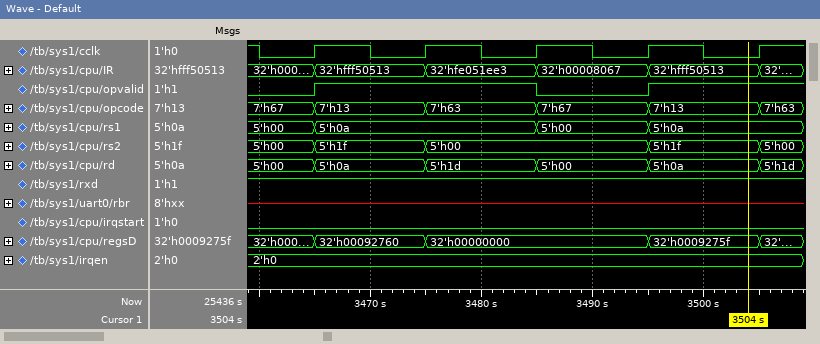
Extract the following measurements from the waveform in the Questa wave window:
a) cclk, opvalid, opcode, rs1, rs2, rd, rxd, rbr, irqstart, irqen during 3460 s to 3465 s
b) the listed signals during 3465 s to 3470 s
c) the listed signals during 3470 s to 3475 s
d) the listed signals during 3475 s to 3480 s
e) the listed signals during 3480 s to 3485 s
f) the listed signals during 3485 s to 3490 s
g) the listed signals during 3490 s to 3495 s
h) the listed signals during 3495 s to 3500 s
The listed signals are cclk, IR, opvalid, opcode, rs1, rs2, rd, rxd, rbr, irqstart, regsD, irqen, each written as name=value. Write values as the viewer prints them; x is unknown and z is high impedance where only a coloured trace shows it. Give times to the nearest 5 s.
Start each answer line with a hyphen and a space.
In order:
- cclk=0, opvalid=0, opcode=7'h67, rs1=5'h00, rs2=5'h00, rd=5'h00, rxd=1, rbr=x, irqstart=0, irqen=2'h0
- cclk=1, IR=32'hfff50513, opvalid=1, opcode=7'h13, rs1=5'h0a, rs2=5'h1f, rd=5'h0a, rxd=1, rbr=x, irqstart=0, regsD=32'h00092760, irqen=2'h0
- cclk=0, IR=32'hfff50513, opvalid=1, opcode=7'h13, rs1=5'h0a, rs2=5'h1f, rd=5'h0a, rxd=1, rbr=x, irqstart=0, regsD=32'h00092760, irqen=2'h0
- cclk=1, IR=32'hfe051ee3, opvalid=1, opcode=7'h63, rs1=5'h0a, rs2=5'h00, rd=5'h1d, rxd=1, rbr=x, irqstart=0, regsD=32'h00000000, irqen=2'h0
- cclk=0, IR=32'hfe051ee3, opvalid=1, opcode=7'h63, rs1=5'h0a, rs2=5'h00, rd=5'h1d, rxd=1, rbr=x, irqstart=0, regsD=32'h00000000, irqen=2'h0
- cclk=1, IR=32'h00008067, opvalid=0, opcode=7'h67, rs1=5'h00, rs2=5'h00, rd=5'h00, rxd=1, rbr=x, irqstart=0, regsD=32'h00000000, irqen=2'h0
- cclk=0, IR=32'h00008067, opvalid=0, opcode=7'h67, rs1=5'h00, rs2=5'h00, rd=5'h00, rxd=1, rbr=x, irqstart=0, regsD=32'h00000000, irqen=2'h0
- cclk=1, IR=32'hfff50513, opvalid=1, opcode=7'h13, rs1=5'h0a, rs2=5'h1f, rd=5'h0a, rxd=1, rbr=x, irqstart=0, regsD=32'h0009275f, irqen=2'h0
